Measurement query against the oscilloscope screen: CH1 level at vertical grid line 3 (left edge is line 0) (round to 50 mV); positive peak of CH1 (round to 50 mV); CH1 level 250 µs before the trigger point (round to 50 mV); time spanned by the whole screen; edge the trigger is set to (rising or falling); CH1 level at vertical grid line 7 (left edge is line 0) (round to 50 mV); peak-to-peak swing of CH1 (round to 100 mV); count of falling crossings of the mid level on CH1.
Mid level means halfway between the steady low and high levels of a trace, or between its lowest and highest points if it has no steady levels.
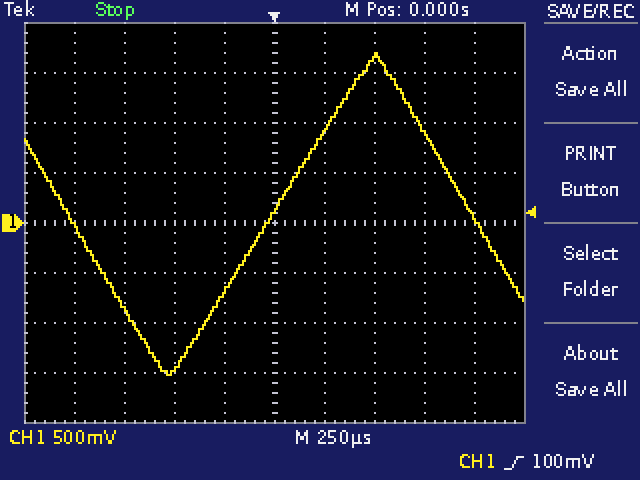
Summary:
-1.50 V
1.70 V
-700 mV
2.5 ms
rising
1.65 V
3.20 V
2
